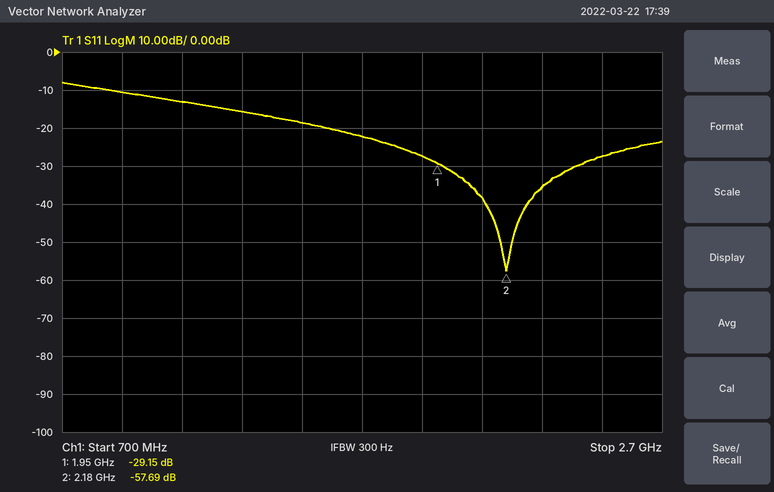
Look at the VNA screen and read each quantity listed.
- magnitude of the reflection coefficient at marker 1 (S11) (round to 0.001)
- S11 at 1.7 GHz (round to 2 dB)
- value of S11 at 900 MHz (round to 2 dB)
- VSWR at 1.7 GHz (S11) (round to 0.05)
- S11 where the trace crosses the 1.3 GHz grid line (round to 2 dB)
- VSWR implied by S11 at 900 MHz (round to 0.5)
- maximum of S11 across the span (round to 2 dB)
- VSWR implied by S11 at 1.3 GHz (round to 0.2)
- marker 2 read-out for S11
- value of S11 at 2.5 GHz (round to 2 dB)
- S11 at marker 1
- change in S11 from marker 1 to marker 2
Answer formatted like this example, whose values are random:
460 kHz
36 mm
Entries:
0.035
-22 dB
-10 dB
1.15
-16 dB
2.0
-8 dB
1.4
-57.69 dB
-28 dB
-29.15 dB
-28.54 dB
